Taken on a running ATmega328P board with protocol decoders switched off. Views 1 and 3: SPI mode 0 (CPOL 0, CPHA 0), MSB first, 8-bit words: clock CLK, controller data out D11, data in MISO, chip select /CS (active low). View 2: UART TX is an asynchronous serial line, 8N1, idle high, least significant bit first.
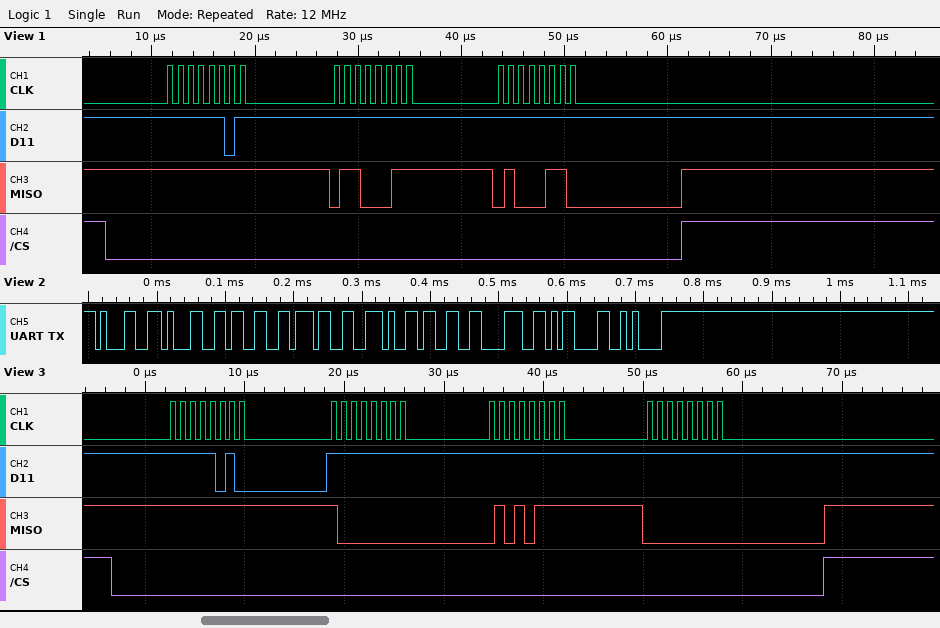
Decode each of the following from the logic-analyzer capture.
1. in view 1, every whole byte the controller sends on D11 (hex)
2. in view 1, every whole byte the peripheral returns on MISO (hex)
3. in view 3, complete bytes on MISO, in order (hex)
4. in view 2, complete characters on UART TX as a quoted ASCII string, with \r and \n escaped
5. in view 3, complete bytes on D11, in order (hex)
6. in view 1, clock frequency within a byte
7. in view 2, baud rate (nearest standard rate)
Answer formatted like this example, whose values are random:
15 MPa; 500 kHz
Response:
FD FF FF; FF 63 46; 0xFF 0x80 0x57 0x00; "1137.38\r\n"; 0xFA 0xFF 0xFF 0xFF; 1 MHz; 115200 baud
